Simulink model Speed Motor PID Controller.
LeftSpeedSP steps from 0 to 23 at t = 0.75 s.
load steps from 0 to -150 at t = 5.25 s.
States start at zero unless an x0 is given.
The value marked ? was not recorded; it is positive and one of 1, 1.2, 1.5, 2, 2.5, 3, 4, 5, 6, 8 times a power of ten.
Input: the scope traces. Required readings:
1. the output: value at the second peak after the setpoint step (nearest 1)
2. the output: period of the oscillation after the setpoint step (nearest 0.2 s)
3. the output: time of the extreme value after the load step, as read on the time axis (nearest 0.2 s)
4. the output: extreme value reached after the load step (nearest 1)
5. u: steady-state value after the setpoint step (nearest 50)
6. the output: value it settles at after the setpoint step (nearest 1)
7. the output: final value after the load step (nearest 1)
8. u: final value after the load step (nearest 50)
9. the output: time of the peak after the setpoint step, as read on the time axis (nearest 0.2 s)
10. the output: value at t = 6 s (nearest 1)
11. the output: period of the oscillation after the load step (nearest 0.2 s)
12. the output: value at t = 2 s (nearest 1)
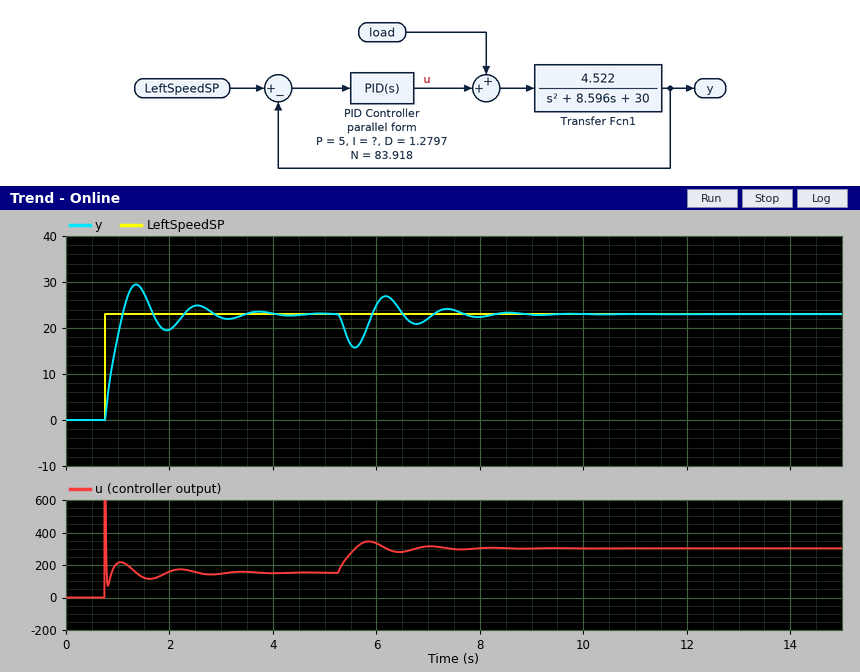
25
1.2 s
5.6 s
16
150
23
23
300
1.4 s
25
1.2 s
20
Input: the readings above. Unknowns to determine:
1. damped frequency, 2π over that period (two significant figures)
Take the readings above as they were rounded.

5.2 rad/s
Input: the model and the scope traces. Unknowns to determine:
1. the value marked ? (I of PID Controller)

80
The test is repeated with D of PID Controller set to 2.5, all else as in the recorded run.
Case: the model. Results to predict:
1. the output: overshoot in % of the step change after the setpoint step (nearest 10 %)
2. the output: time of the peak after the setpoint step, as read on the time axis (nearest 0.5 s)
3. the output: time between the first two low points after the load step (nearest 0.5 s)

20 %
1.5 s
1.5 s
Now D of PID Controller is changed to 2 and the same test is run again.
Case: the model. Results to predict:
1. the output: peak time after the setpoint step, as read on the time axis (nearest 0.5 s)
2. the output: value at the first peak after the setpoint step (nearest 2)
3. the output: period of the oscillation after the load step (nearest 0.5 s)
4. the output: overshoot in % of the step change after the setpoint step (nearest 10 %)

1.5 s
28
1.5 s
20 %
